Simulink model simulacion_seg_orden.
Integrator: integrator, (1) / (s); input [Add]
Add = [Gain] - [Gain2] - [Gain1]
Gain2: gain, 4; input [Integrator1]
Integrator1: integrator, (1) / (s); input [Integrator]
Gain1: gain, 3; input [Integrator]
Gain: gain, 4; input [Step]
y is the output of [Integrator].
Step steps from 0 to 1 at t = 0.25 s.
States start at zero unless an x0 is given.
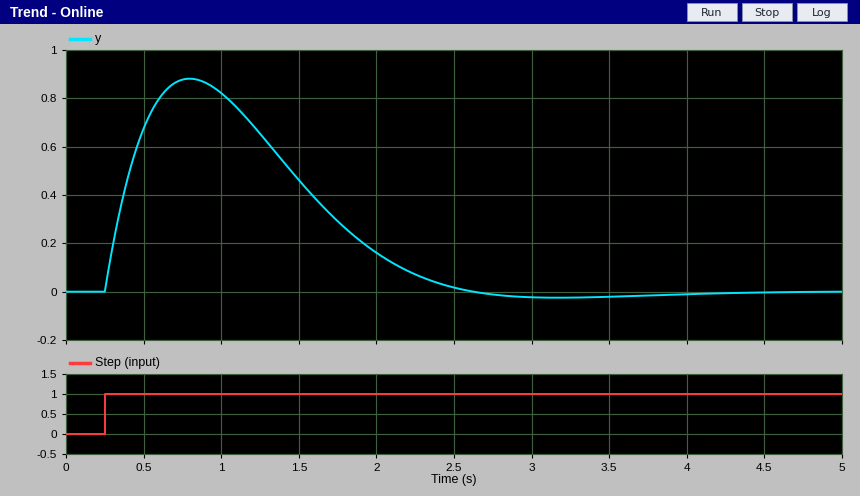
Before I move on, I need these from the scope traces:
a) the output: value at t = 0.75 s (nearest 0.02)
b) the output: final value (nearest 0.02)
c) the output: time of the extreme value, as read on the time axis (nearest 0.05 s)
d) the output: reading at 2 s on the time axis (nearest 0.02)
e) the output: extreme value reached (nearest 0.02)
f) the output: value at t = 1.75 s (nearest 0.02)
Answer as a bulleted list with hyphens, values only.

- 0.88
- 0.00
- 0.80 s
- 0.16
- 0.88
- 0.30
